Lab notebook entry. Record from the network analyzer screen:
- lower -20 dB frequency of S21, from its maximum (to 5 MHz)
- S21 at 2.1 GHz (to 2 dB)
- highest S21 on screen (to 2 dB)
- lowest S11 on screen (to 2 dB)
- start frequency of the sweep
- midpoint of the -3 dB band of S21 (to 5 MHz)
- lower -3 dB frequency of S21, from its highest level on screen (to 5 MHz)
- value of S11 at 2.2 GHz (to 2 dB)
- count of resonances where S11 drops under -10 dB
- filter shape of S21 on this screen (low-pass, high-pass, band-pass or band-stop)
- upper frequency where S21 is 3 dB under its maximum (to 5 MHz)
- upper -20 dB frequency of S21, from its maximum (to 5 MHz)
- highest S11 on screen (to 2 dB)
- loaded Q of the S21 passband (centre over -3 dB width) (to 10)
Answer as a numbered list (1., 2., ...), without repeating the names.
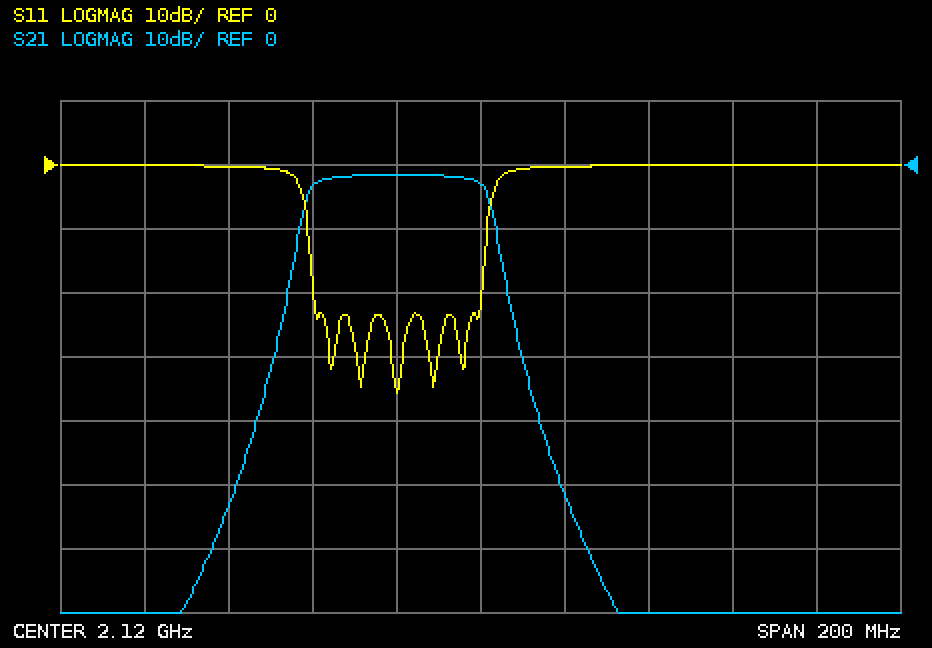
1. 2.075 GHz
2. -2 dB
3. -2 dB
4. -36 dB
5. 2.02 GHz
6. 2.100 GHz
7. 2.080 GHz
8. 0 dB
9. 5
10. band-pass
11. 2.120 GHz
12. 2.125 GHz
13. 0 dB
14. 50
